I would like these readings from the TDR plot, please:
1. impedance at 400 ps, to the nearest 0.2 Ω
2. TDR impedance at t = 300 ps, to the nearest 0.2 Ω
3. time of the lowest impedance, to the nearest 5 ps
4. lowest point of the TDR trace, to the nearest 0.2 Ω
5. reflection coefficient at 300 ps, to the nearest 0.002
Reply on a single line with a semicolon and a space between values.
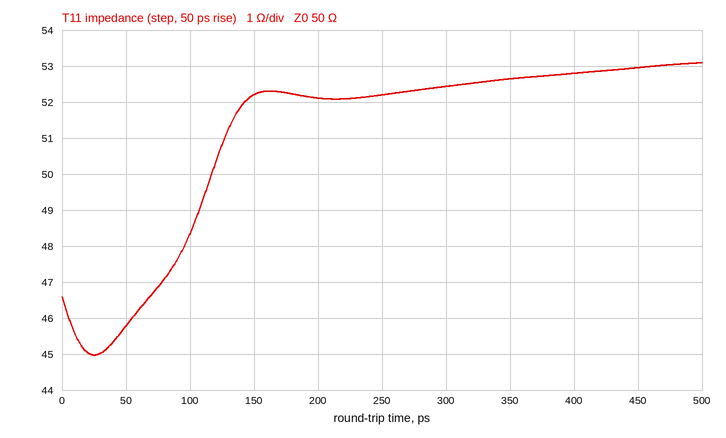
52.8 Ω; 52.4 Ω; 25 ps; 45.0 Ω; +0.024
